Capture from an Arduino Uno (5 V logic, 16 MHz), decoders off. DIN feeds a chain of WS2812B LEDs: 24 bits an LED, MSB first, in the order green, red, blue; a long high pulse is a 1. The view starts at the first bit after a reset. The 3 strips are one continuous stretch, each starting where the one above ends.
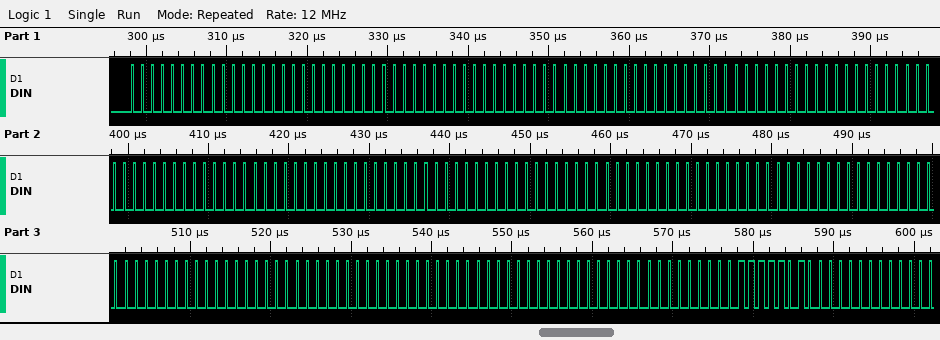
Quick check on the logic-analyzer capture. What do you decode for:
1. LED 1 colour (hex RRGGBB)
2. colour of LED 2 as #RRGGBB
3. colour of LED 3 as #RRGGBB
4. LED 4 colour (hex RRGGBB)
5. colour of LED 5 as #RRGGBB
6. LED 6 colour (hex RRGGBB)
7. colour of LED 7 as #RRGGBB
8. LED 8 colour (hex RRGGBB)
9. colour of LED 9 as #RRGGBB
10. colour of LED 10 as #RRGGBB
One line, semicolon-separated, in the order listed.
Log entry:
#000000; #000000; #000000; #000000; #000000; #000000; #000000; #000000; #000000; #FA0000
